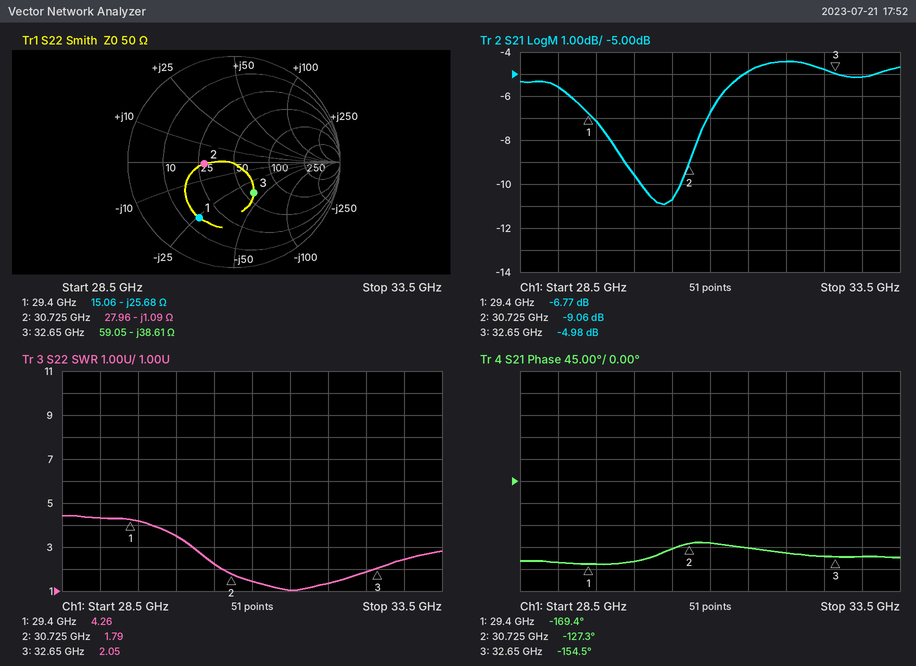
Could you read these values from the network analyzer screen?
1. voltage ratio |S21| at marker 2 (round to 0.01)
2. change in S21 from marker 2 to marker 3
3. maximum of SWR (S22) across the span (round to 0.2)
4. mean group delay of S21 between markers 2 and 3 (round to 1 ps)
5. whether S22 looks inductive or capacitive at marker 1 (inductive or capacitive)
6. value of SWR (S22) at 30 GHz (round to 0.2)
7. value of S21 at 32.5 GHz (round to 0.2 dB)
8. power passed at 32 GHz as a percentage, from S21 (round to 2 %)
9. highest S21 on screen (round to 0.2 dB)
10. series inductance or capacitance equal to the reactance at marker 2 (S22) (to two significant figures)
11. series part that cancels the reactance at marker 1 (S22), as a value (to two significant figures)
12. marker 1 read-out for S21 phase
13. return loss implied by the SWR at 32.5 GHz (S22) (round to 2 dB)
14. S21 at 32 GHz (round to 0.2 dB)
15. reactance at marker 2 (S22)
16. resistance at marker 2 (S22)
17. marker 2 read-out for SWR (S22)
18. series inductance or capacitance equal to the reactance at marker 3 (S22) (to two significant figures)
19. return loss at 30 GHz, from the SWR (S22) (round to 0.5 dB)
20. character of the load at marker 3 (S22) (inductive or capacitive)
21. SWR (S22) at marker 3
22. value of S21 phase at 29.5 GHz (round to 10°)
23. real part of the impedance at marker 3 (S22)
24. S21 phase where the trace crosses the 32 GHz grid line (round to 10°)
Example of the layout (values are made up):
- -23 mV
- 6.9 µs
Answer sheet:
- 0.35
- 4.08 dB
- 4.4
- 39 ps
- capacitive
- 3.6
- -4.8 dB
- 36 %
- -4.4 dB
- 4.8 pF
- 140 pH
- -169.4°
- 10 dB
- -4.4 dB
- -1.09 Ω
- 27.96 Ω
- 1.79
- 130 fF
- 5.0 dB
- capacitive
- 2.05
- -170°
- 59.05 Ω
- -150°
